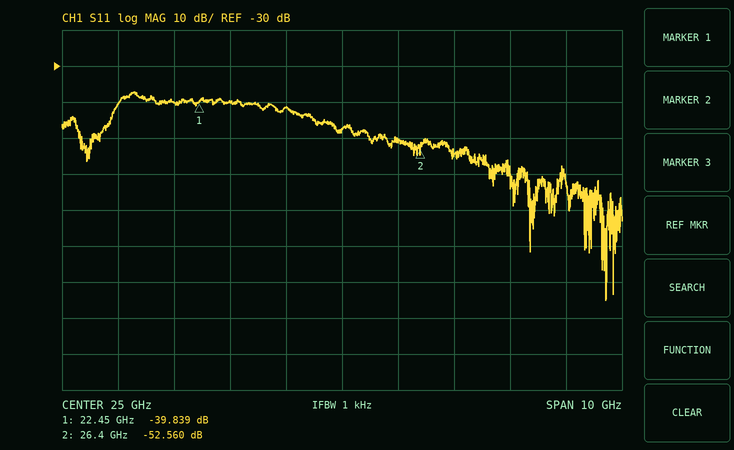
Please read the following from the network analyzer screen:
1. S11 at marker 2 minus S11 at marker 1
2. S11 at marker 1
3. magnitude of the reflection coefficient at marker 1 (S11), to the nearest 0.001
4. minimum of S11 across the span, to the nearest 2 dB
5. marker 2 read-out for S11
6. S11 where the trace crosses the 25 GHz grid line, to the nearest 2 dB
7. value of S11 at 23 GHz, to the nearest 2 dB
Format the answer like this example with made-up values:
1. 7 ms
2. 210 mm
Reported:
1. -12.721 dB
2. -39.839 dB
3. 0.010
4. -96 dB
5. -52.560 dB
6. -48 dB
7. -40 dB
